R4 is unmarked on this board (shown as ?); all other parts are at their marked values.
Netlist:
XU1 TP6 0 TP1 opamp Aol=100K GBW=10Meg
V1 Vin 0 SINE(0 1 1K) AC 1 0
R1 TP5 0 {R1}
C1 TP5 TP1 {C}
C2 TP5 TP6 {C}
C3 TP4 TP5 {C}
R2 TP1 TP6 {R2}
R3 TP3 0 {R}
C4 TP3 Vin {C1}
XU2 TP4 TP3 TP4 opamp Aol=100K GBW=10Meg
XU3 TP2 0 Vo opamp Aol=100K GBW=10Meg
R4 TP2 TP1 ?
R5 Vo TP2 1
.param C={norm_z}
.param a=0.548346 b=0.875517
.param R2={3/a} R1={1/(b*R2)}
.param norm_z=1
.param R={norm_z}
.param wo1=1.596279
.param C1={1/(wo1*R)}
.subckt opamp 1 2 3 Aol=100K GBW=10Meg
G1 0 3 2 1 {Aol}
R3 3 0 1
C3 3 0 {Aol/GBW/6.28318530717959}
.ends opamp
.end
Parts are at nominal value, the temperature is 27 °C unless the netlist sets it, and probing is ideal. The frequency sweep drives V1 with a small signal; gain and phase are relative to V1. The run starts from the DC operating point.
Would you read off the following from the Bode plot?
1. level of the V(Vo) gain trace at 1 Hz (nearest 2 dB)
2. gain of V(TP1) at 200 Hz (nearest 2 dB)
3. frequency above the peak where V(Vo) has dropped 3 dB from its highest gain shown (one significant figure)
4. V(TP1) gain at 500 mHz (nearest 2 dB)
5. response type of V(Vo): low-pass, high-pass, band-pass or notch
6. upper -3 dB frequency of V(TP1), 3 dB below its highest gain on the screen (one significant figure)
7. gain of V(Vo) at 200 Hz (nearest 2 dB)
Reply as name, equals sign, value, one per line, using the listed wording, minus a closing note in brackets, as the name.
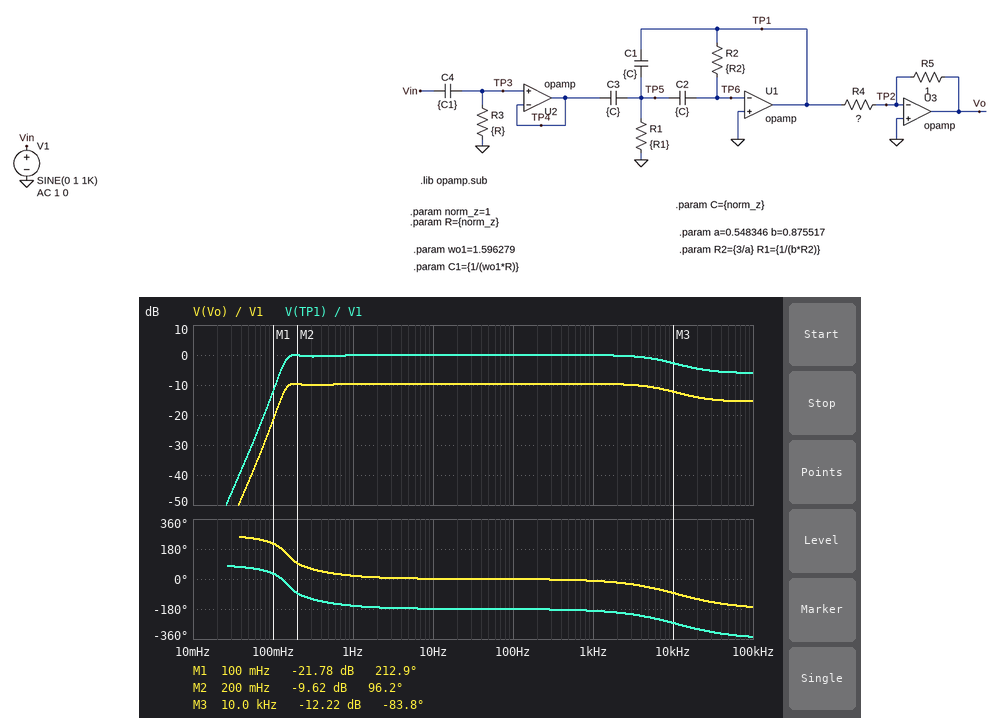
level of the V(Vo) gain trace at 1 Hz = -10 dB
gain of V(TP1) at 200 Hz = 0 dB
frequency above the peak where V(Vo) has dropped 3 dB from its highest gain shown = 10 kHz
V(TP1) gain at 500 mHz = 0 dB
response type of V(Vo): low-pass, high-pass, band-pass or notch = high-pass
upper -3 dB frequency of V(TP1), 3 dB below its highest gain on the screen = 10 kHz
gain of V(Vo) at 200 Hz = -10 dB
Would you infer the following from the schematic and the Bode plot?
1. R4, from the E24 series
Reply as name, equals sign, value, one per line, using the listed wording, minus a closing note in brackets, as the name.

R4, from the E24 series = 3 Ω
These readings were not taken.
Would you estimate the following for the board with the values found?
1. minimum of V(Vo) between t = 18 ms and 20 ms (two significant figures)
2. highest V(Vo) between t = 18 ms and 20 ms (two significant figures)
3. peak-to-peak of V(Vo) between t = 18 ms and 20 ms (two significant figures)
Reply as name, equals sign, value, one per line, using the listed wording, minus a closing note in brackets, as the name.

minimum of V(Vo) between t = 18 ms and 20 ms = -330 mV
highest V(Vo) between t = 18 ms and 20 ms = 330 mV
peak-to-peak of V(Vo) between t = 18 ms and 20 ms = 660 mV
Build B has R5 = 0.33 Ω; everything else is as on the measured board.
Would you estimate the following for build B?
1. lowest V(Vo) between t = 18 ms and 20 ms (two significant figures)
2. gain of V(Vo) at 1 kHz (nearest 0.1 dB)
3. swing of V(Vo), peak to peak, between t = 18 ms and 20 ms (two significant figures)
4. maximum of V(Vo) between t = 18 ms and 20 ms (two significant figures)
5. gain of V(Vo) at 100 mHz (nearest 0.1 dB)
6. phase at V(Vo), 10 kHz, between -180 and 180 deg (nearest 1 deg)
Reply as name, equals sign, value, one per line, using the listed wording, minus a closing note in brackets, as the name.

lowest V(Vo) between t = 18 ms and 20 ms = -110 mV
gain of V(Vo) at 1 kHz = -19.2 dB
swing of V(Vo), peak to peak, between t = 18 ms and 20 ms = 220 mV
maximum of V(Vo) between t = 18 ms and 20 ms = 110 mV
gain of V(Vo) at 100 mHz = -31.4 dB
phase at V(Vo), 10 kHz, between -180 and 180 deg = -84 deg
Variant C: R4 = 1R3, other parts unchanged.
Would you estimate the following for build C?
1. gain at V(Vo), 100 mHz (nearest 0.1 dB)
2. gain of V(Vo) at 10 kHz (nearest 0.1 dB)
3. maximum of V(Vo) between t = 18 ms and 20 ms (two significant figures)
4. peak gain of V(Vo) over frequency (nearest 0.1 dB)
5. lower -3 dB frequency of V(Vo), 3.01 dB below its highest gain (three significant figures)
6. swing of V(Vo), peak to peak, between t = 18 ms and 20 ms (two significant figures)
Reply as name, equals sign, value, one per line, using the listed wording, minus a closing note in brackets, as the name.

gain at V(Vo), 100 mHz = -14.5 dB
gain of V(Vo) at 10 kHz = -5.0 dB
maximum of V(Vo) between t = 18 ms and 20 ms = 760 mV
peak gain of V(Vo) over frequency = -2.3 dB
lower -3 dB frequency of V(Vo), 3.01 dB below its highest gain = 136 mHz
swing of V(Vo), peak to peak, between t = 18 ms and 20 ms = 1.5 V
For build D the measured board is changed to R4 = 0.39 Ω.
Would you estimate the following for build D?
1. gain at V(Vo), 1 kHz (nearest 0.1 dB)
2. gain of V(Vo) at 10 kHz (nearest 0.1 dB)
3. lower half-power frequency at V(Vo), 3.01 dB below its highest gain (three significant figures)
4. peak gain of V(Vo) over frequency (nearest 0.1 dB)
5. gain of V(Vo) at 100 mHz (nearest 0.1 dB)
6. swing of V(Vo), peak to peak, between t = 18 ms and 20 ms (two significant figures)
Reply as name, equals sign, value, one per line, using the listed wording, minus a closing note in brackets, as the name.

gain at V(Vo), 1 kHz = 8.1 dB
gain of V(Vo) at 10 kHz = 5.5 dB
lower half-power frequency at V(Vo), 3.01 dB below its highest gain = 136 mHz
peak gain of V(Vo) over frequency = 8.2 dB
gain of V(Vo) at 100 mHz = -4.1 dB
swing of V(Vo), peak to peak, between t = 18 ms and 20 ms = 5.1 V
